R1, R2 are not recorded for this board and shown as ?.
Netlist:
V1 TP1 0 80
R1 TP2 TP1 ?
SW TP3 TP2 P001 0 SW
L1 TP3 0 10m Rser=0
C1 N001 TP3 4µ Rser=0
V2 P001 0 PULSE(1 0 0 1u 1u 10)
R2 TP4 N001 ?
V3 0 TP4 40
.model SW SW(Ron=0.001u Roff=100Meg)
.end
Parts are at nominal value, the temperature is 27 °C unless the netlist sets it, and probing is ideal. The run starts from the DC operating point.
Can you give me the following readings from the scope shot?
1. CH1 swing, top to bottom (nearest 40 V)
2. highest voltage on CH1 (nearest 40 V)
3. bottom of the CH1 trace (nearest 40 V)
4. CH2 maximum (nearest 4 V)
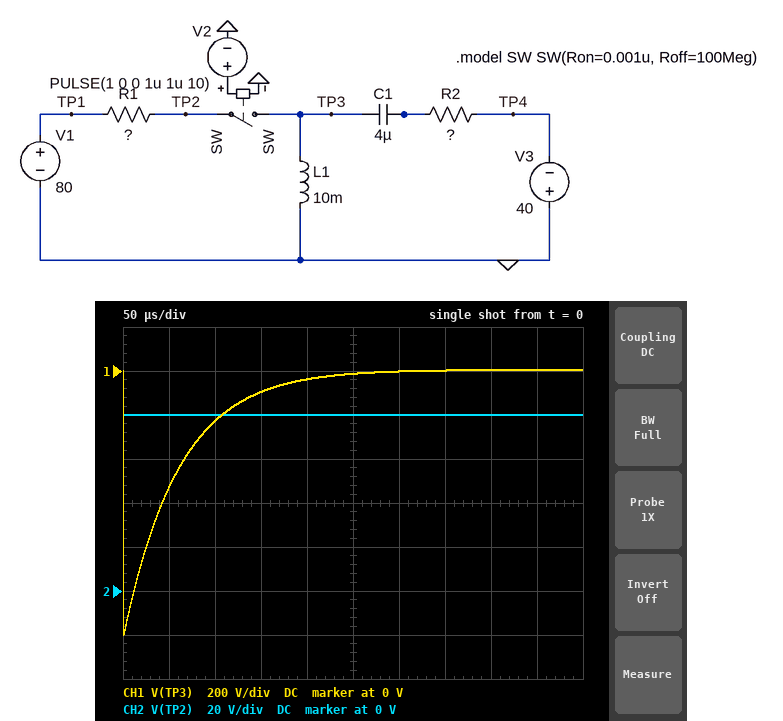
1.20 kV
0 V
-1.20 kV
80 V
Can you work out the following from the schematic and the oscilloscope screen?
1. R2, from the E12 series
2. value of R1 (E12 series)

180 Ω
12 Ω
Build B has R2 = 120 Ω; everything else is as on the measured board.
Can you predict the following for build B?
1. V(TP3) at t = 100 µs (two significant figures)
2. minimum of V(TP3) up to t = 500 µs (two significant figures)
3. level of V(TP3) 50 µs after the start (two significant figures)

-290 V
-800 V
-490 V
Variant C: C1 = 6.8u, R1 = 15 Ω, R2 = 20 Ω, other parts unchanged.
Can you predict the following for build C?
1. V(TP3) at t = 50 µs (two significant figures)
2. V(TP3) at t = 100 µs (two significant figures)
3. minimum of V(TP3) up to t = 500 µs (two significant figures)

-130 V
-150 V
-170 V
